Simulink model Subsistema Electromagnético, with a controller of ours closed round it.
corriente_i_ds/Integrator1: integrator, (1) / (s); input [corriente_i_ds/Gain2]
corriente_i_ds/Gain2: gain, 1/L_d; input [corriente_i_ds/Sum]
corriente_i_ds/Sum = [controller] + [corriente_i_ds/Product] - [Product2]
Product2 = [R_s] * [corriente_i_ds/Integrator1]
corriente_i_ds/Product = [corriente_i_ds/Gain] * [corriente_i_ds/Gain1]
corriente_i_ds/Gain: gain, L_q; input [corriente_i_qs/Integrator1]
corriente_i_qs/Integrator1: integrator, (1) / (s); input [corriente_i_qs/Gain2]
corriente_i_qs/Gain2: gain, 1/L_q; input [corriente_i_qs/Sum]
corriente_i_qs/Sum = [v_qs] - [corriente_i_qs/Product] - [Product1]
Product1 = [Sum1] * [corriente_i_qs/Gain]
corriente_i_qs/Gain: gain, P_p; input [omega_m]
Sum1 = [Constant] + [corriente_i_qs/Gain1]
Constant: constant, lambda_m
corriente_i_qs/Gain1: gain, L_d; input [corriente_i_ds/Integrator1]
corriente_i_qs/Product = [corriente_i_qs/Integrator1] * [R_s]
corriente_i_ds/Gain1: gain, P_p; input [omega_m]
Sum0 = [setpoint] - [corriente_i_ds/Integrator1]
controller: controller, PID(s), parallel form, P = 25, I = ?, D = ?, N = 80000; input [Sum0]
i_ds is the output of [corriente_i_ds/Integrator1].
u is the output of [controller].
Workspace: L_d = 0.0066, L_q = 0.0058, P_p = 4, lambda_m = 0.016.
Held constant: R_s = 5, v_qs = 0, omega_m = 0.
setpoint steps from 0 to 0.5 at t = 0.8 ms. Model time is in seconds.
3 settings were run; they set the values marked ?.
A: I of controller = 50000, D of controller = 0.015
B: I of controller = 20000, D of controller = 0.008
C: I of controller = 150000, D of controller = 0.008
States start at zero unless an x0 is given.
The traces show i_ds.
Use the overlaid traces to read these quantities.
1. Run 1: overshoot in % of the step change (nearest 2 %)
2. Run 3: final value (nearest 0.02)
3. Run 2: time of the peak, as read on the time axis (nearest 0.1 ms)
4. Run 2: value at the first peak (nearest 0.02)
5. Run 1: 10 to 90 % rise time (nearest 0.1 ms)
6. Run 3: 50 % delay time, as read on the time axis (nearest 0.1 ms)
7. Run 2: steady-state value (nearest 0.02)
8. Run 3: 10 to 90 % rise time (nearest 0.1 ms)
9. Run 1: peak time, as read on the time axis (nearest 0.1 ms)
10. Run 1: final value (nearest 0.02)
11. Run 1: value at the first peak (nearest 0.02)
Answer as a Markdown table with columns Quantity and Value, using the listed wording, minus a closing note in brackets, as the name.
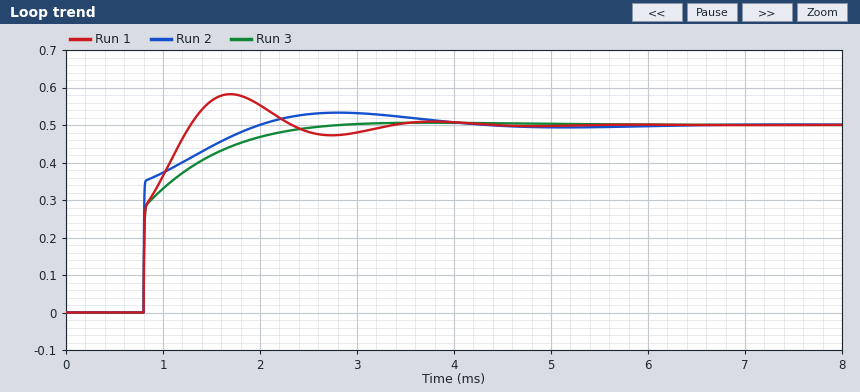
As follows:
| Quantity | Value |
|---|---|
| Run 1: overshoot in % of the step change | 16 % |
| Run 3: final value | 0.50 |
| Run 2: time of the peak, as read on the time axis | 2.8 ms |
| Run 2: value at the first peak | 0.54 |
| Run 1: 10 to 90 % rise time | 0.4 ms |
| Run 3: 50 % delay time, as read on the time axis | 0.8 ms |
| Run 2: steady-state value | 0.50 |
| Run 3: 10 to 90 % rise time | 1.0 ms |
| Run 1: peak time, as read on the time axis | 1.7 ms |
| Run 1: final value | 0.50 |
| Run 1: value at the first peak | 0.58 |
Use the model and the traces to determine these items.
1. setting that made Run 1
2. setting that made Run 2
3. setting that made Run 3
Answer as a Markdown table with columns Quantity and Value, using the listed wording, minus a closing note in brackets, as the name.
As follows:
| Quantity | Value |
|---|---|
| setting that made Run 1 | C |
| setting that made Run 2 | A |
| setting that made Run 3 | B |
